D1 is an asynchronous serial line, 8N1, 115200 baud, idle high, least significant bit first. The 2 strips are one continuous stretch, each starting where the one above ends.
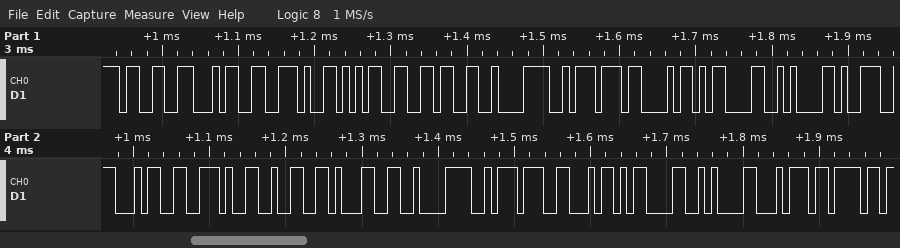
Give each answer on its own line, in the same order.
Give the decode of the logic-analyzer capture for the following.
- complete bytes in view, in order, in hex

33 34 2E 35 36 C2 BA 43 0D 0A 39 34 2E 32 31 C2 BA 46 0D 0A 74 6F
